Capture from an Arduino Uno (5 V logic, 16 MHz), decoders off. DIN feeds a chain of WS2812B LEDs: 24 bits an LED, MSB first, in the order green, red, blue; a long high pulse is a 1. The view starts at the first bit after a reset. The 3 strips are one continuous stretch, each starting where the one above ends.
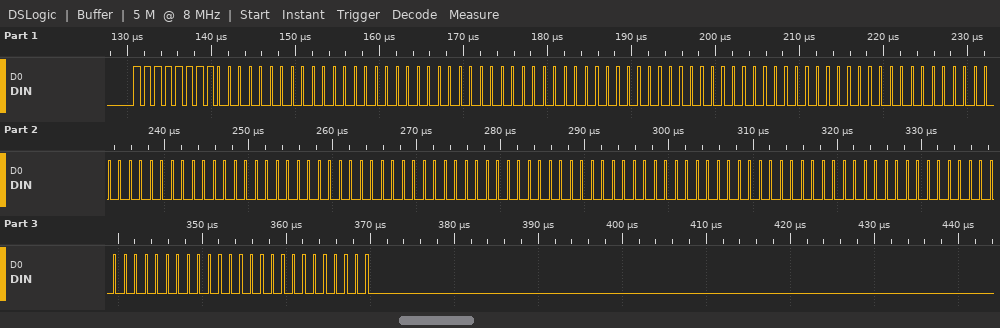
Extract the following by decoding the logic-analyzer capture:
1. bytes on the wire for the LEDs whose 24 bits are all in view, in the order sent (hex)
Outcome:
FF 00 00 00 00 00 00 00 00 00 00 00 00 00 00 00 00 00 00 00 00 00 00 00
